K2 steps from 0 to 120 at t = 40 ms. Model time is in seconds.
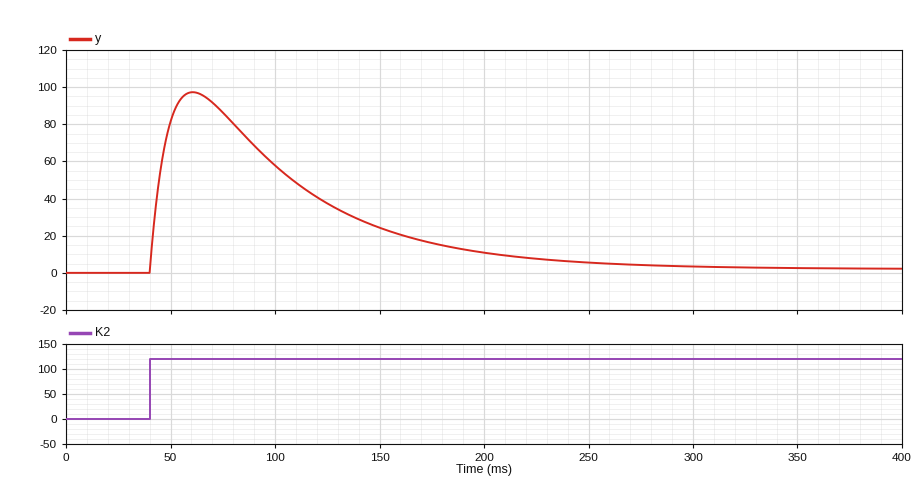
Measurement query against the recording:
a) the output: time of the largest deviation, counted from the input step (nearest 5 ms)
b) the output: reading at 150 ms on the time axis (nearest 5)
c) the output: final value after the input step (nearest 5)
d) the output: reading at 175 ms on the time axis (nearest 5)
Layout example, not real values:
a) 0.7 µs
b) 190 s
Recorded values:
a) 20 ms
b) 25
c) 0
d) 15
